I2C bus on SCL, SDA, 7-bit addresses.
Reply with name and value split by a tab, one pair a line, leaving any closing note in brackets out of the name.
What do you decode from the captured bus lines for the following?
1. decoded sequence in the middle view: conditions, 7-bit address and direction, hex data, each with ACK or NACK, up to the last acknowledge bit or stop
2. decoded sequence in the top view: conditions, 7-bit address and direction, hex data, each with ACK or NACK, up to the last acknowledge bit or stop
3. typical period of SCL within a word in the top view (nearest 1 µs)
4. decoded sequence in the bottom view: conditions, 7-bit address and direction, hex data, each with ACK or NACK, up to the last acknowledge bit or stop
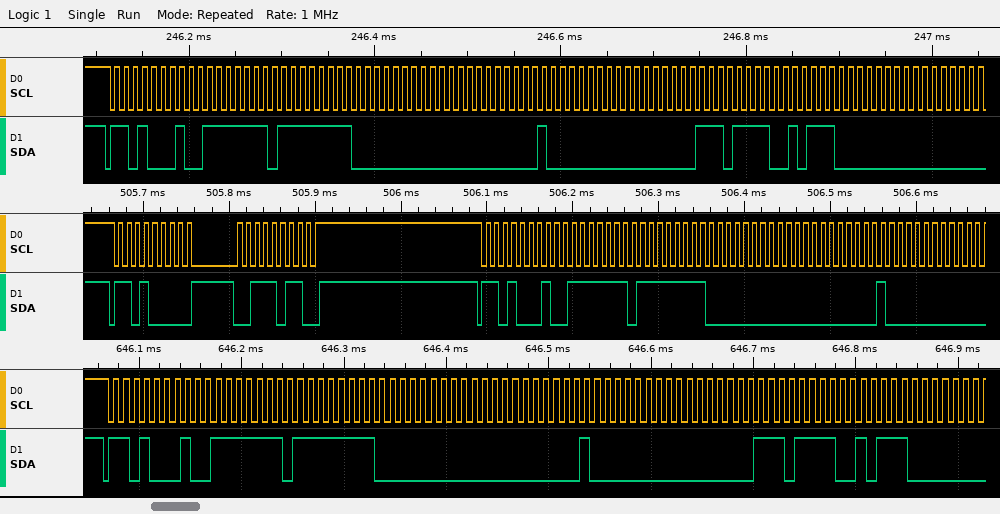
decoded sequence in the middle view: conditions, 7-bit address and direction, hex data, each with ACK or NACK, up to the last acknowledge bit or stop	start, address 68 write ACK, 3B ACK, stop, start, address 68 read ACK, 7F ACK, FF ACK, 00 ACK, 00 ACK, 40 ACK
decoded sequence in the top view: conditions, 7-bit address and direction, hex data, each with ACK or NACK, up to the last acknowledge bit or stop	start, address 68 read ACK, 7F ACK, FF ACK, 00 ACK, 00 ACK, 40 ACK, 00 ACK, EF ACK, 5C ACK, 00 ACK
typical period of SCL within a word in the top view	10 µs
decoded sequence in the bottom view: conditions, 7-bit address and direction, hex data, each with ACK or NACK, up to the last acknowledge bit or stop	start, address 68 read ACK, 7F ACK, FF ACK, 00 ACK, 00 ACK, 40 ACK, 00 ACK, EF ACK, 5C ACK
